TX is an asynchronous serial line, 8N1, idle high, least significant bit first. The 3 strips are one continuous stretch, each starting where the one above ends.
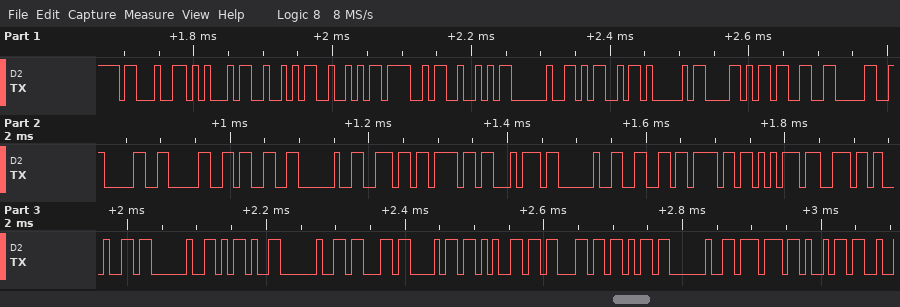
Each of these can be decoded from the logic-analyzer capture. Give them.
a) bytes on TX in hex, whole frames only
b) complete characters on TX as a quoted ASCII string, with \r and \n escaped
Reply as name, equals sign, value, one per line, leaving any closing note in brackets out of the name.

bytes on TX in hex, whole frames only = 0x23 0x45 0x52 0x52 0x4F 0x52 0x20 0x4D 0x41 0x58 0x33 0x30 0x30 0x30 0x33 0x20 0x6E 0x6F 0x74 0x20 0x66 0x6F 0x75 0x6E 0x64 0x20 0x2D 0x20 0x63 0x68 0x65 0x63 0x6B 0x20 0x77 0x69
complete characters on TX as a quoted ASCII string, with \r and \n escaped = "#ERROR MAX30003 not found - check wi"
